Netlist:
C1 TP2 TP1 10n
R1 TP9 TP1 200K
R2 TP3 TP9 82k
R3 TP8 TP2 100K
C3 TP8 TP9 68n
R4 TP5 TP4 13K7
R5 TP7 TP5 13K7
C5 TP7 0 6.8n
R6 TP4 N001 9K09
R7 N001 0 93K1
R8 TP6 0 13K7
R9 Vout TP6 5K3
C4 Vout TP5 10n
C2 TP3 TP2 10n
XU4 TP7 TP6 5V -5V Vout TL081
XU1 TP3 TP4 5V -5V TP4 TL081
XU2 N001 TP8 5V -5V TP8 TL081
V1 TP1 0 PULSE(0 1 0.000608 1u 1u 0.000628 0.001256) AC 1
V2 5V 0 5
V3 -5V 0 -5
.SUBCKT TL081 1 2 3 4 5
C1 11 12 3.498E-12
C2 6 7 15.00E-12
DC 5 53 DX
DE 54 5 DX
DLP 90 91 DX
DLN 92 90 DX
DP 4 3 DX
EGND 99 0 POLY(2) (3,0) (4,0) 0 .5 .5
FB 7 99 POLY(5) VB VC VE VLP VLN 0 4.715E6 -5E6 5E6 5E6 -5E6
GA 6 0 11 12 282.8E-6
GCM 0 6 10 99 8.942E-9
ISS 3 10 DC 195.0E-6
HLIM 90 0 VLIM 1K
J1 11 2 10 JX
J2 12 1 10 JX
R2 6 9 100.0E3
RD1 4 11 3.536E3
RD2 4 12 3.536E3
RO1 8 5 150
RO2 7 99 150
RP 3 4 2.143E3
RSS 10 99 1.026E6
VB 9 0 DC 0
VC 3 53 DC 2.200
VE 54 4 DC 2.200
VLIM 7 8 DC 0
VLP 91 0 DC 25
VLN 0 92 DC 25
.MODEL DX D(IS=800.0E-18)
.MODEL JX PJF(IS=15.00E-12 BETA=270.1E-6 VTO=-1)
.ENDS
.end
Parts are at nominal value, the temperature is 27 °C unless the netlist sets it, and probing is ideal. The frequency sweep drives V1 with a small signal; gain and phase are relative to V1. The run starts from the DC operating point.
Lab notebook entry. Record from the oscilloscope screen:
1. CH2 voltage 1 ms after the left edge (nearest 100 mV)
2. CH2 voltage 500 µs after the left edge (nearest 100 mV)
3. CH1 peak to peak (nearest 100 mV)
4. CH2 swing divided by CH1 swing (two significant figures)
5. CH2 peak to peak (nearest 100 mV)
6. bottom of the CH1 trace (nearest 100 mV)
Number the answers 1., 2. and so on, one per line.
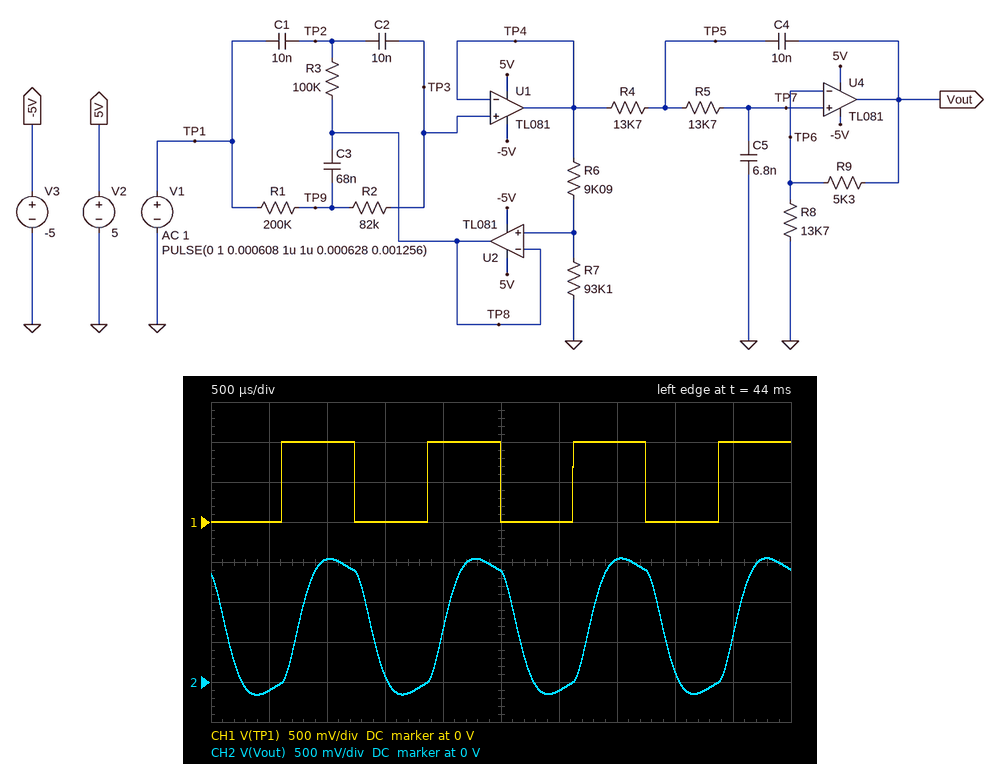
1. 1.5 V
2. -100 mV
3. 1.0 V
4. 1.7
5. 1.7 V
6. 0 V
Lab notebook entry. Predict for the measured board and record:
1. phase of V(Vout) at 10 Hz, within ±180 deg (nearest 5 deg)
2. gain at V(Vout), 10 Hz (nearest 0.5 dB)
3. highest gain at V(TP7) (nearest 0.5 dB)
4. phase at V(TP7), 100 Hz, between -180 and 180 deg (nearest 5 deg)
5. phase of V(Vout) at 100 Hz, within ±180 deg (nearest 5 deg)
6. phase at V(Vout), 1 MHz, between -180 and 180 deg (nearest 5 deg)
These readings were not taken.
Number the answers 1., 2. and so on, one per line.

1. -5 deg
2. 3.0 dB
3. 0.5 dB
4. 60 deg
5. 60 deg
6. 60 deg
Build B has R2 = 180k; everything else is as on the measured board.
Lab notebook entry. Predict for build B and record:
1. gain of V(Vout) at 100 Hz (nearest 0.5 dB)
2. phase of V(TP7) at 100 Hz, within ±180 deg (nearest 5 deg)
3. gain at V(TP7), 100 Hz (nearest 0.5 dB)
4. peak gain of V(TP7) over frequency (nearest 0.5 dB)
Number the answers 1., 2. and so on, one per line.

1. 3.5 dB
2. 20 deg
3. 0.5 dB
4. 12.5 dB
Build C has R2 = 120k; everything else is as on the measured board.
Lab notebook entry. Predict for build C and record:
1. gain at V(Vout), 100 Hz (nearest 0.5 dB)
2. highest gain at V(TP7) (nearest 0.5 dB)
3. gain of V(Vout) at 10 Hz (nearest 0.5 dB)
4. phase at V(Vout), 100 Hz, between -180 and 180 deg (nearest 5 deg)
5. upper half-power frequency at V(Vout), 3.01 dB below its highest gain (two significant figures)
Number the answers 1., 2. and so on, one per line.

1. 3.5 dB
2. 4.0 dB
3. 3.0 dB
4. 35 deg
5. 90 Hz
